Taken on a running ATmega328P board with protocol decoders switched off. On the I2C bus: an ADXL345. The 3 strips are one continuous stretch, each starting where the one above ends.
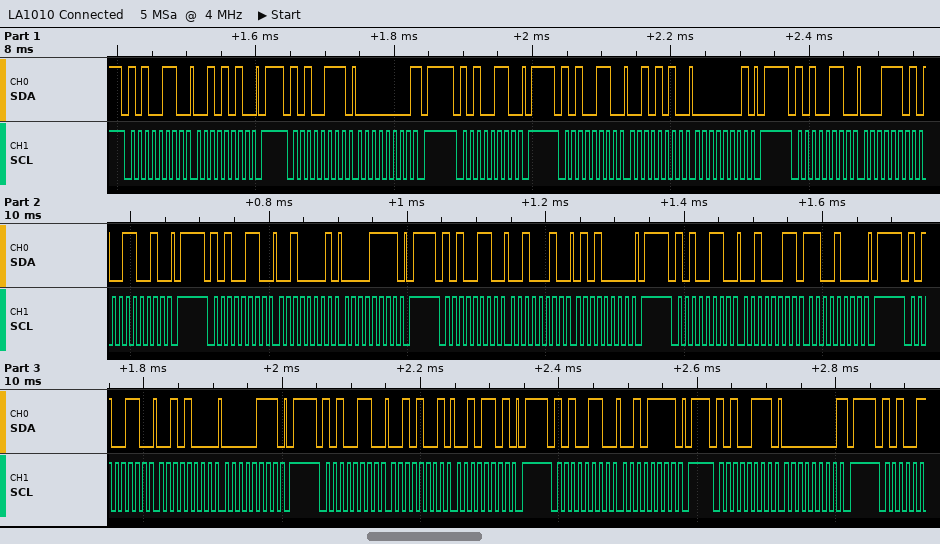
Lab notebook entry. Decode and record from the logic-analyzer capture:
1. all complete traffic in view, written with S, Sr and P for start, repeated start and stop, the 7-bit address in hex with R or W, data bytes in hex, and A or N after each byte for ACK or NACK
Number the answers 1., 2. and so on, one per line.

1. S 53W A 2A A P S 53R A 00 N P S 53W A P S 53W A 2A A 01 A P S 53W A 1D A 32 A P S 53W A 21 A 0F A P S 53W A 22 A 50 A P S 53W A 23 A C8 A P S 53W A 28 A 07 A P S 53W A 29 A 2D A P S 53W A 2F A P S 53R A 00 N P
